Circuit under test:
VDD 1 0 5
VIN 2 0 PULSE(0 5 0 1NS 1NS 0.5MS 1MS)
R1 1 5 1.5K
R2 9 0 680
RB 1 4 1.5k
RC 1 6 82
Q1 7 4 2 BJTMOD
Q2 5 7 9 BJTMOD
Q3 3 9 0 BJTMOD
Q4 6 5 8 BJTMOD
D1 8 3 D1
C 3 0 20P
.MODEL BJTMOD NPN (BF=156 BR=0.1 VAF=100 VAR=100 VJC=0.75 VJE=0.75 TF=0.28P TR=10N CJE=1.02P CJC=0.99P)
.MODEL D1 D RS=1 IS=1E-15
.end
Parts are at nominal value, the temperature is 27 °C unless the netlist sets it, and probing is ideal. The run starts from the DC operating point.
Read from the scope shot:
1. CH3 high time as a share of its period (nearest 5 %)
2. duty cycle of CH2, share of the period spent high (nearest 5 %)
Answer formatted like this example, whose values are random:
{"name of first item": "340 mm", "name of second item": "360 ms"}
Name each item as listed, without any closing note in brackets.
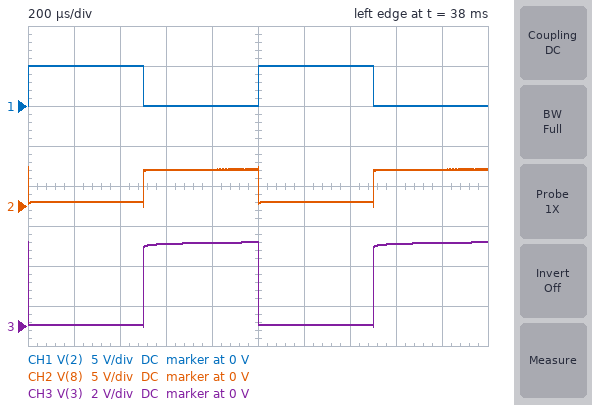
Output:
{"CH3 high time as a share of its period": "50 %", "duty cycle of CH2, share of the period spent high": "50 %"}
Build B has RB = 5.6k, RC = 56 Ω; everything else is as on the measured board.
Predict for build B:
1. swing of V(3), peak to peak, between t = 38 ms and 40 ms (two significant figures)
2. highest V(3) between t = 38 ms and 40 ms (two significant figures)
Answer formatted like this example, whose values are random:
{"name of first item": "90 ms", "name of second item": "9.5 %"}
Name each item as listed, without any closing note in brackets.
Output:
{"swing of V(3), peak to peak, between t = 38 ms and 40 ms": "4.2 V", "highest V(3) between t = 38 ms and 40 ms": "4.2 V"}
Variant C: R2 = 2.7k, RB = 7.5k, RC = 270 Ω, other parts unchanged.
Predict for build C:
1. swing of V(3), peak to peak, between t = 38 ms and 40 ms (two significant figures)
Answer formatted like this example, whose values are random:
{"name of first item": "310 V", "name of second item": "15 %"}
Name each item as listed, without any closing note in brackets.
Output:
{"swing of V(3), peak to peak, between t = 38 ms and 40 ms": "4.2 V"}
